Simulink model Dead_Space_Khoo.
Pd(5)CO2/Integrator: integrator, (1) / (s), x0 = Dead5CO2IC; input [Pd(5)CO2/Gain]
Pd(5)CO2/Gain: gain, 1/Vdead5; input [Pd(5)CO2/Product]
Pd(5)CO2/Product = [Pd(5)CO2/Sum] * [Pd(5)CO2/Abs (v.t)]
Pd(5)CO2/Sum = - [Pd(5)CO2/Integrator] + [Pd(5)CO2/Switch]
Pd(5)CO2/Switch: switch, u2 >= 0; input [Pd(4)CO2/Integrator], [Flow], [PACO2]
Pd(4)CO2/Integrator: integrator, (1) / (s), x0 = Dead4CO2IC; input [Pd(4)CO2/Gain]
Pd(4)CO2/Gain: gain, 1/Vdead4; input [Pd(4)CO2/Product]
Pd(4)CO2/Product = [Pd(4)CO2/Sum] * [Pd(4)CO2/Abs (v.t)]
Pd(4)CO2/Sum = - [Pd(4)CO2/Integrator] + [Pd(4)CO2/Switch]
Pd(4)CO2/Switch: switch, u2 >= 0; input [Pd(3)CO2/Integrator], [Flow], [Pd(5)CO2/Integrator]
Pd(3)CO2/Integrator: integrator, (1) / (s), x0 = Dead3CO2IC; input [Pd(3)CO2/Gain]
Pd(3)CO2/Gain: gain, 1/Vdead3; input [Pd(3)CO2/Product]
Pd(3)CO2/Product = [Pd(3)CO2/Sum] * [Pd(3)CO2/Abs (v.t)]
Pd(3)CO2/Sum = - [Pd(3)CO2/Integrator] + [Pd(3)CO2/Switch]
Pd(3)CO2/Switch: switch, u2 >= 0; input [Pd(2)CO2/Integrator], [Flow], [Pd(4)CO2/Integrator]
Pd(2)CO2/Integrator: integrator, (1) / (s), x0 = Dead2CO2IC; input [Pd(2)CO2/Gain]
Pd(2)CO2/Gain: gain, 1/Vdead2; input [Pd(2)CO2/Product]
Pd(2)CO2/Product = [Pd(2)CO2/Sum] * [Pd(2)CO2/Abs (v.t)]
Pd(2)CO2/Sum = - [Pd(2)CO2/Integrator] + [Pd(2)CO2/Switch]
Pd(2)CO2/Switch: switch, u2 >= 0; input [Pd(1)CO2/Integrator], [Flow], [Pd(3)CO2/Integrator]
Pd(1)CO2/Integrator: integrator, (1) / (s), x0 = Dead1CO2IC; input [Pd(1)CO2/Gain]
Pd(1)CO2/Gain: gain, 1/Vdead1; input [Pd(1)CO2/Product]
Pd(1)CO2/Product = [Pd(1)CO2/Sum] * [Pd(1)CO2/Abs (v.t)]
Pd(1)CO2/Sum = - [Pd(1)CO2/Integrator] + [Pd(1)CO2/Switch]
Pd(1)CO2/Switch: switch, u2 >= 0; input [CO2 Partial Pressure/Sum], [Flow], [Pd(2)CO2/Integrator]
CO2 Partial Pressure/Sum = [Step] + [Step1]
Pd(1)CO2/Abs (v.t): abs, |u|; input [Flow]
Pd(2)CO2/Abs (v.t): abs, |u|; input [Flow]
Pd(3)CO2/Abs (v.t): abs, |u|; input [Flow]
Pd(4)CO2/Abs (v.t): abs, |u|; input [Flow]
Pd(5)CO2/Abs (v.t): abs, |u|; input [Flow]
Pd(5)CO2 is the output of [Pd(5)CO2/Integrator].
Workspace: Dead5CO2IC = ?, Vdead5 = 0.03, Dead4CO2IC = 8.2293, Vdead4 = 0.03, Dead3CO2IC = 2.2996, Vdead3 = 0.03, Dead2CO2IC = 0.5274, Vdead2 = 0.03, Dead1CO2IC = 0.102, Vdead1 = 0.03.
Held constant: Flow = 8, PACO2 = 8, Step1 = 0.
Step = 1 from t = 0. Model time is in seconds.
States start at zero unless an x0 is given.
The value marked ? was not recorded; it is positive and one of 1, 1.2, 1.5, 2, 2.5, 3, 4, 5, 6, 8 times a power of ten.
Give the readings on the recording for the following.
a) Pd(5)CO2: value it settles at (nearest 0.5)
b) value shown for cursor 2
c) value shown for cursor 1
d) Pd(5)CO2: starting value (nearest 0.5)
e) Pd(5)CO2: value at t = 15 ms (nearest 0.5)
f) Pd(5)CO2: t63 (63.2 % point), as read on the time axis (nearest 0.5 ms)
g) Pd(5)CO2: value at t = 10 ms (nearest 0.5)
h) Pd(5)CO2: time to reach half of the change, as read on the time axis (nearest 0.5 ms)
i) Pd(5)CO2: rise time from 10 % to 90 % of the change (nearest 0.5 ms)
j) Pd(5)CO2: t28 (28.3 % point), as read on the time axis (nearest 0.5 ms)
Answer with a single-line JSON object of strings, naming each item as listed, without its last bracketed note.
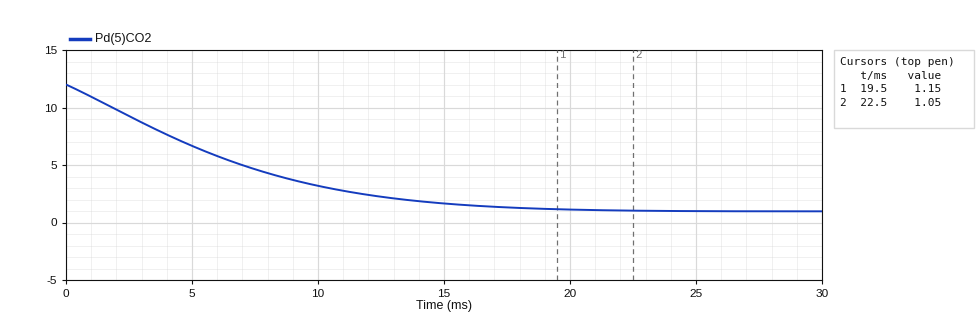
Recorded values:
{"Pd(5)CO2: value it settles at": "1.0", "value shown for cursor 2": "1.05", "value shown for cursor 1": "1.15", "Pd(5)CO2: starting value": "12.0", "Pd(5)CO2: value at t = 15 ms": "1.5", "Pd(5)CO2: t63 (63.2 % point), as read on the time axis": "7.0 ms", "Pd(5)CO2: value at t = 10 ms": "3.0", "Pd(5)CO2: time to reach half of the change, as read on the time axis": "5.0 ms", "Pd(5)CO2: rise time from 10 % to 90 % of the change": "12.0 ms", "Pd(5)CO2: t28 (28.3 % point), as read on the time axis": "3.0 ms"}
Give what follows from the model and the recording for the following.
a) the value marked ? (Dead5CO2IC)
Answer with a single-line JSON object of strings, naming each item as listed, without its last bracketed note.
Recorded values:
{"the value marked ?": "12"}
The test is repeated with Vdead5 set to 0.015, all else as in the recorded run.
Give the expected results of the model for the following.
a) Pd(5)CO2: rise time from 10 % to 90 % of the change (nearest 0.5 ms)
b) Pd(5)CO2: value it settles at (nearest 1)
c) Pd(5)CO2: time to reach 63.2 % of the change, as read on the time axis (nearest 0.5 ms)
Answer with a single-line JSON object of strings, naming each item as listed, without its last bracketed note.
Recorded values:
{"Pd(5)CO2: rise time from 10 % to 90 % of the change": "9.0 ms", "Pd(5)CO2: value it settles at": "1", "Pd(5)CO2: time to reach 63.2 % of the change, as read on the time axis": "5.0 ms"}
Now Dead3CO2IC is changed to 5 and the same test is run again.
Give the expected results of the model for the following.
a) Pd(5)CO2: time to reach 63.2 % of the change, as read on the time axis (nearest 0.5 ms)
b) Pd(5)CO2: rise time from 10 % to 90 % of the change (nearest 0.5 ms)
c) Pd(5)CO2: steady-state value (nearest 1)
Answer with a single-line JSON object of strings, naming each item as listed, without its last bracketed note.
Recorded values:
{"Pd(5)CO2: time to reach 63.2 % of the change, as read on the time axis": "8.0 ms", "Pd(5)CO2: rise time from 10 % to 90 % of the change": "13.5 ms", "Pd(5)CO2: steady-state value": "1"}
